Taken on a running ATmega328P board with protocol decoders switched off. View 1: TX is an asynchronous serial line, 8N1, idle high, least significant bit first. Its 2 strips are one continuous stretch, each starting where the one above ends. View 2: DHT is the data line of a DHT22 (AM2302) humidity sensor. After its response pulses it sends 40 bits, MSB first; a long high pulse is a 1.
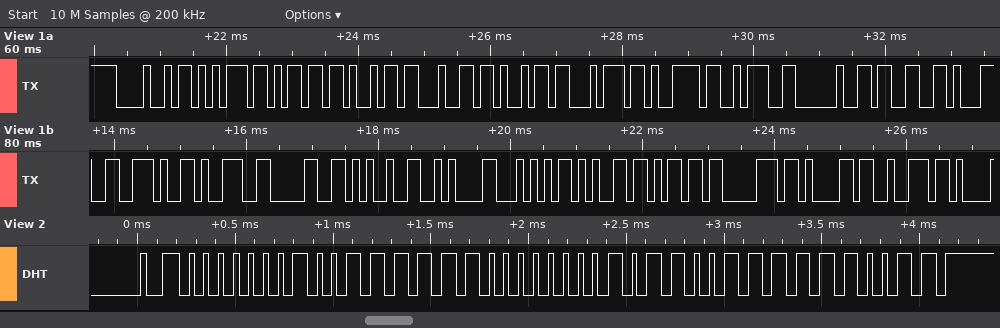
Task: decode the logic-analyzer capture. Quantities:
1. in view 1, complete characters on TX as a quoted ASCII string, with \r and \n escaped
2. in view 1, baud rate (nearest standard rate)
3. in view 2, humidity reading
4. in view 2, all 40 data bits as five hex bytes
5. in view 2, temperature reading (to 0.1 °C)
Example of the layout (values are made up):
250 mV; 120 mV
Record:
"Humidity: 31.90%\nTempar"; 9600 baud; 31.9 %; 01 3F 00 B3 F3; 17.9 °C
